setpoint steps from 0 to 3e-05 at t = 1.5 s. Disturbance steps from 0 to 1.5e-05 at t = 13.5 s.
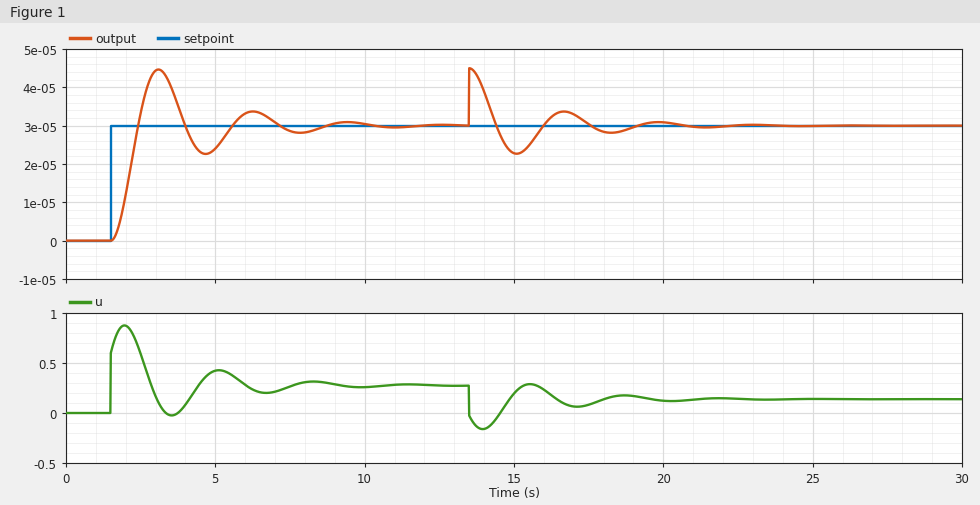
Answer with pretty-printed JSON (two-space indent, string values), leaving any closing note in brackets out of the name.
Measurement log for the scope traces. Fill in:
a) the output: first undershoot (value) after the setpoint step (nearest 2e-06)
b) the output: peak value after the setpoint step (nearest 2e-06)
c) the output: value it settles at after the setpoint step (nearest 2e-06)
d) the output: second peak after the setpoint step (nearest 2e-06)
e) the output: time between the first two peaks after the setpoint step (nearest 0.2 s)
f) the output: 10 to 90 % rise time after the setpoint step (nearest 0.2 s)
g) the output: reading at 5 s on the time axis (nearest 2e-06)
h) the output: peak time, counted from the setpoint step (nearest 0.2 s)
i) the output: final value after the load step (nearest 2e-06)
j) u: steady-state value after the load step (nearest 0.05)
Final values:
{
  "the output: first undershoot (value) after the setpoint step": "0.000022",
  "the output: peak value after the setpoint step": "0.000044",
  "the output: value it settles at after the setpoint step": "0.000030",
  "the output: second peak after the setpoint step": "0.000034",
  "the output: time between the first two peaks after the setpoint step": "3.2 s",
  "the output: 10 to 90 % rise time after the setpoint step": "0.6 s",
  "the output: reading at 5 s on the time axis": "0.000024",
  "the output: peak time, counted from the setpoint step": "1.6 s",
  "the output: final value after the load step": "0.000030",
  "u: steady-state value after the load step": "0.15"
}
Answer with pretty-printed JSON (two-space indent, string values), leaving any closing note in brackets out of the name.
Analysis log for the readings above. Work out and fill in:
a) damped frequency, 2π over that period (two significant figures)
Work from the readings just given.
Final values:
{
  "damped frequency, 2π over that period": "2.0 rad/s"
}
